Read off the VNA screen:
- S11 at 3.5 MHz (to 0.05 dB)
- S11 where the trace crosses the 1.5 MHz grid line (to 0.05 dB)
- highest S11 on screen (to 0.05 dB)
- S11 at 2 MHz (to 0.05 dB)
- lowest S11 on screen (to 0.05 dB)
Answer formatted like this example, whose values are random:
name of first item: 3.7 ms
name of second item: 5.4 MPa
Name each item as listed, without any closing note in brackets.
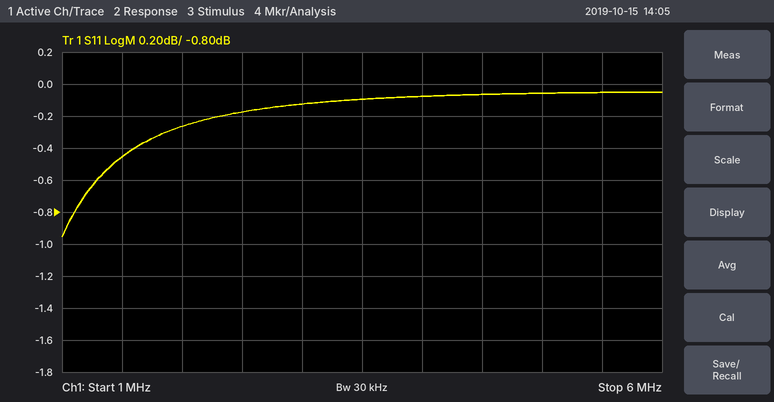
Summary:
S11 at 3.5 MHz: -0.10 dB
S11 where the trace crosses the 1.5 MHz grid line: -0.45 dB
highest S11 on screen: -0.05 dB
S11 at 2 MHz: -0.25 dB
lowest S11 on screen: -0.95 dB
